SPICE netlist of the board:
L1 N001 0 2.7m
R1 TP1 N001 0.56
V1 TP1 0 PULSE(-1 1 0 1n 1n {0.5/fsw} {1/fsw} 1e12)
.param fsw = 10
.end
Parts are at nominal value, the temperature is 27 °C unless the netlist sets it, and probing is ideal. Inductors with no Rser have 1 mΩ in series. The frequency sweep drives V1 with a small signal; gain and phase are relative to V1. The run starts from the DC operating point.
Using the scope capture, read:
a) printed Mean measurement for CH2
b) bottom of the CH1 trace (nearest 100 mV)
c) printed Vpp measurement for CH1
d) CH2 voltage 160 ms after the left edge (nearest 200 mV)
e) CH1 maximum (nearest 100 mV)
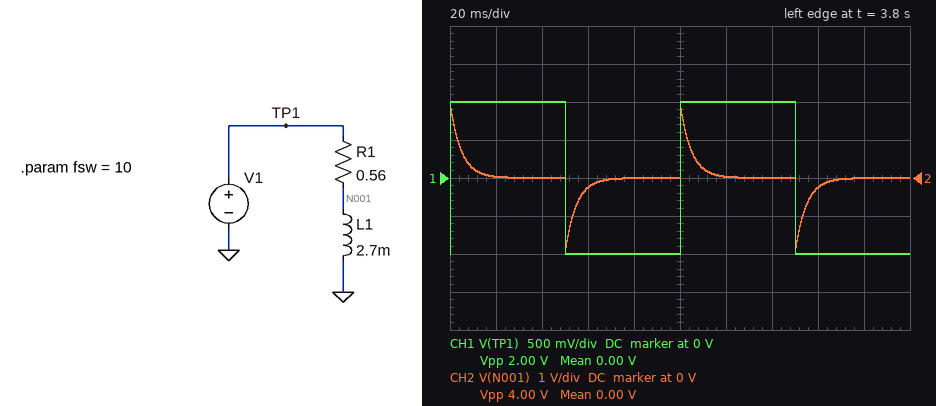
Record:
0.00 V
-1.0 V
2.00 V
-200 mV
1.0 V
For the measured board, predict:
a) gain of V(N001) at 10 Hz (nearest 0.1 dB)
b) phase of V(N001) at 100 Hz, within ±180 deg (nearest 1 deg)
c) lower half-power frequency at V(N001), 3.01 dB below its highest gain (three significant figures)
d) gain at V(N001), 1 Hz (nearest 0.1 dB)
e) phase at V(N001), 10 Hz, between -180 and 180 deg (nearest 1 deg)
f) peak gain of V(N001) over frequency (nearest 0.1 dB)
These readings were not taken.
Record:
-10.8 dB
18 deg
33.1 Hz
-30.4 dB
73 deg
0 dB
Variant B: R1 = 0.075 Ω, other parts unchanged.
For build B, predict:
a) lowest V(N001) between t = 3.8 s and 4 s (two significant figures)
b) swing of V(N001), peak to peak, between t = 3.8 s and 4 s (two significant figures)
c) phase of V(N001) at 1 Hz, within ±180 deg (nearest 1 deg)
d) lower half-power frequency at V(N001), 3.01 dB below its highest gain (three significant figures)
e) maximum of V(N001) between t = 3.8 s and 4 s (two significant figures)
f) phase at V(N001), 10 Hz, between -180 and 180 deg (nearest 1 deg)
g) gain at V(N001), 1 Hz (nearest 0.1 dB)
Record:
-1.6 V
3.2 V
74 deg
4.48 Hz
1.6 V
24 deg
-13.2 dB
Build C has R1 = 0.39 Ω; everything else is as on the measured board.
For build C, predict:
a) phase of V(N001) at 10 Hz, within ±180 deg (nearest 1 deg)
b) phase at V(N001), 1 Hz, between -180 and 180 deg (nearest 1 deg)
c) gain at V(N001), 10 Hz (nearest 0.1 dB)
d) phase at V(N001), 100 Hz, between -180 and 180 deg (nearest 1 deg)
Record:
66 deg
84 deg
-8.0 dB
13 deg
